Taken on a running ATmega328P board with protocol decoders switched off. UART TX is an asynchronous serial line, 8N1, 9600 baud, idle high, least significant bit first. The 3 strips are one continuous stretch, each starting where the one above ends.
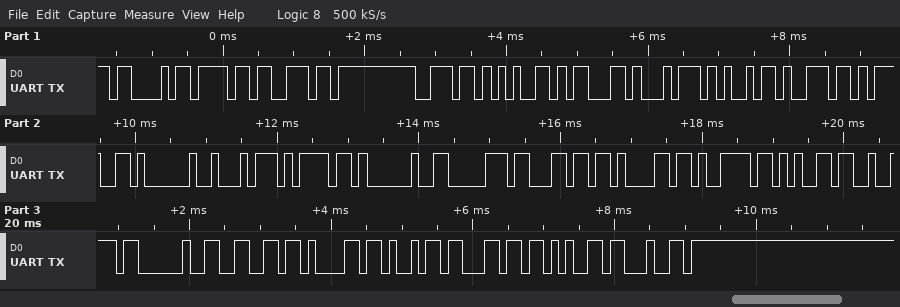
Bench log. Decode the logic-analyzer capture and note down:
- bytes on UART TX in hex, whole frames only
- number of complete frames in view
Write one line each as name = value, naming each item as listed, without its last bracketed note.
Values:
bytes on UART TX in hex, whole frames only = 0x43 0x6F 0x6E 0x6E 0x65 0x63 0x74 0x69 0x6E 0x67 0x20 0x74 0x6F 0x20 0x70 0x6C 0x61 0x79 0x65 0x72 0x20 0x66 0x61 0x69 0x6C 0x65 0x64
number of complete frames in view = 27
